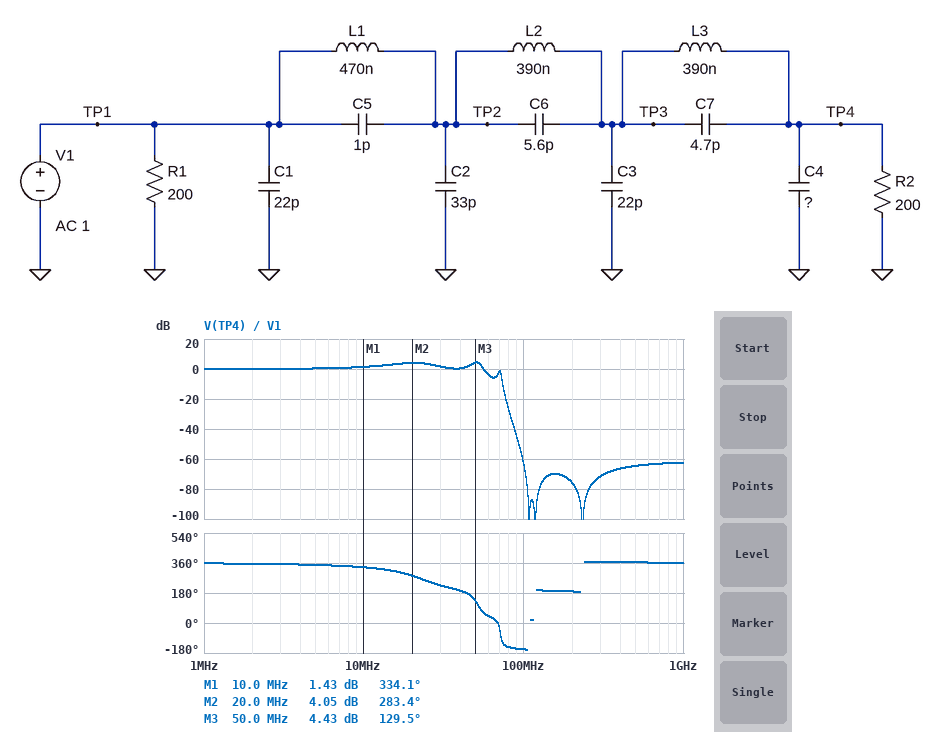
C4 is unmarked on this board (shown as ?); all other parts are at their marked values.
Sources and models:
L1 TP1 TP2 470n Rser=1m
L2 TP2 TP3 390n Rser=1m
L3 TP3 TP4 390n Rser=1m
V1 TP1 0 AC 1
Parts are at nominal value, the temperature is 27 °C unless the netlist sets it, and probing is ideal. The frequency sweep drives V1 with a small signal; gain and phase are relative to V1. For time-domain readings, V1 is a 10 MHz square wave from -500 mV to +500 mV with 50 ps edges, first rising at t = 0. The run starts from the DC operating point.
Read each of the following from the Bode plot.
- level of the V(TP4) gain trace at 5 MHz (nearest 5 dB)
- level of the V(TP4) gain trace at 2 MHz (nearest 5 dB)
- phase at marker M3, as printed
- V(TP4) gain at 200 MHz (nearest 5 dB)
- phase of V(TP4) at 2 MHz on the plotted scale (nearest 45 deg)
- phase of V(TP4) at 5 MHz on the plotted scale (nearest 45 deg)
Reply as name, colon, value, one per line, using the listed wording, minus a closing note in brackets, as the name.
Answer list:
level of the V(TP4) gain trace at 5 MHz: 0 dB
level of the V(TP4) gain trace at 2 MHz: 0 dB
phase at marker M3, as printed: 129.5 deg
V(TP4) gain at 200 MHz: -75 dB
phase of V(TP4) at 2 MHz on the plotted scale: 360 deg
phase of V(TP4) at 5 MHz on the plotted scale: 360 deg
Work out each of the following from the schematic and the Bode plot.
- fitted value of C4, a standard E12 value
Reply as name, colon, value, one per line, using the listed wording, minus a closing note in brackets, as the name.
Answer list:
fitted value of C4, a standard E12 value: 22 pF
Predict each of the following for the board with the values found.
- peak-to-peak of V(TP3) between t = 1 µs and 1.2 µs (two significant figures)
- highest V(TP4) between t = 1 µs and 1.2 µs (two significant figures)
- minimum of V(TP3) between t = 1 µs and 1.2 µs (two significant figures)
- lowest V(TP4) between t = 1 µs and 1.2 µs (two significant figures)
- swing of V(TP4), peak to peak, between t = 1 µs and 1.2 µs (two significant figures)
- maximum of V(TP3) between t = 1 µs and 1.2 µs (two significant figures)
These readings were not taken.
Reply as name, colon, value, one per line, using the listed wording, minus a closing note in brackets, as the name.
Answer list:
peak-to-peak of V(TP3) between t = 1 µs and 1.2 µs: 1.7 V
highest V(TP4) between t = 1 µs and 1.2 µs: 1.0 V
minimum of V(TP3) between t = 1 µs and 1.2 µs: -840 mV
lowest V(TP4) between t = 1 µs and 1.2 µs: -1.0 V
swing of V(TP4), peak to peak, between t = 1 µs and 1.2 µs: 2.1 V
maximum of V(TP3) between t = 1 µs and 1.2 µs: 840 mV
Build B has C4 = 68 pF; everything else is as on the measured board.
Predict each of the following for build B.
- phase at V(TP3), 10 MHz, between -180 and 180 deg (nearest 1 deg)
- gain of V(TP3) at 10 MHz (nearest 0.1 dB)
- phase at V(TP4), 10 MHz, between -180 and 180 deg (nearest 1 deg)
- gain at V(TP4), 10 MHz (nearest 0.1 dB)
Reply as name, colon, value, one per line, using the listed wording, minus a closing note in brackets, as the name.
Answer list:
phase at V(TP3), 10 MHz, between -180 and 180 deg: -26 deg
gain of V(TP3) at 10 MHz: 2.7 dB
phase at V(TP4), 10 MHz, between -180 and 180 deg: -34 deg
gain at V(TP4), 10 MHz: 3.6 dB
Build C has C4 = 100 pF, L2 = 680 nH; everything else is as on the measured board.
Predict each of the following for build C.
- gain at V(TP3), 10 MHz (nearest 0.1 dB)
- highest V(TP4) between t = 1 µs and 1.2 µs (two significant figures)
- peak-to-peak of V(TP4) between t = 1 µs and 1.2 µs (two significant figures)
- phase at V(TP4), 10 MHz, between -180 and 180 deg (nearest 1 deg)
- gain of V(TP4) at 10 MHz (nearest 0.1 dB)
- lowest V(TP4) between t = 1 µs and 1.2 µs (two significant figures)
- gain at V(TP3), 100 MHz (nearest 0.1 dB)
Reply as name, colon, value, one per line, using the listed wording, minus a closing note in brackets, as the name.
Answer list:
gain at V(TP3), 10 MHz: 4.2 dB
highest V(TP4) between t = 1 µs and 1.2 µs: 1.2 V
peak-to-peak of V(TP4) between t = 1 µs and 1.2 µs: 2.4 V
phase at V(TP4), 10 MHz, between -180 and 180 deg: -59 deg
gain of V(TP4) at 10 MHz: 5.5 dB
lowest V(TP4) between t = 1 µs and 1.2 µs: -1.2 V
gain at V(TP3), 100 MHz: -38.2 dB
